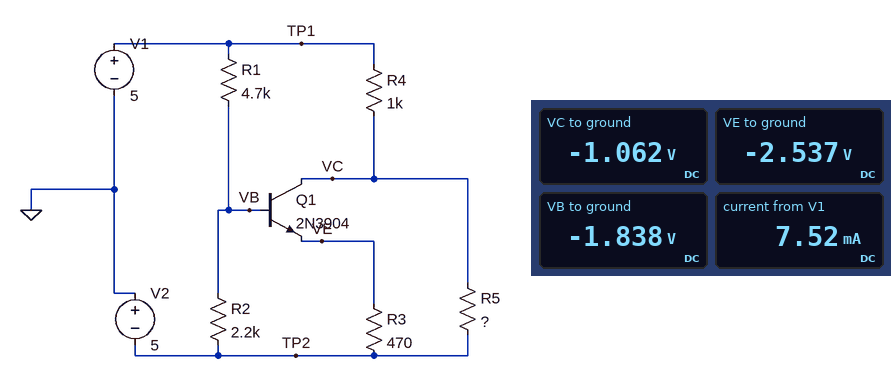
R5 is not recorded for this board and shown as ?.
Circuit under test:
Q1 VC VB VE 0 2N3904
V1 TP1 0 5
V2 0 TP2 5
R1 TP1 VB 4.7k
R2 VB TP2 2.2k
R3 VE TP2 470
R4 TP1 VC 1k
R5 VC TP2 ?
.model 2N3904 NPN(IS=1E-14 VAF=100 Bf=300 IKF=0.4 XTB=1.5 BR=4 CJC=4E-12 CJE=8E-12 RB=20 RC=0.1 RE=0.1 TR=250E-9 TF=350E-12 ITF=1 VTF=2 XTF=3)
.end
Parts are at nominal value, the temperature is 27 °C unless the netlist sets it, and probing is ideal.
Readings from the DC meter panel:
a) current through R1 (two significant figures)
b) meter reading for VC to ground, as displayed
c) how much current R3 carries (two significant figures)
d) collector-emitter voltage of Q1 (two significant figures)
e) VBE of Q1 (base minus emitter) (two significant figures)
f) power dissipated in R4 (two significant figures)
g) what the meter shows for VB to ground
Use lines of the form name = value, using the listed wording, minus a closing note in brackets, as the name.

current through R1 = 1.5 mA
meter reading for VC to ground, as displayed = -1.062 V
how much current R3 carries = 5.2 mA
collector-emitter voltage of Q1 = 1.5 V
VBE of Q1 (base minus emitter) = 700 mV
power dissipated in R4 = 37 mW
what the meter shows for VB to ground = -1.838 V
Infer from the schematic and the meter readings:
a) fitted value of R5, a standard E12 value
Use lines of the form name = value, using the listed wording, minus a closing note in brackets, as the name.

fitted value of R5, a standard E12 value = 4.7 kΩ
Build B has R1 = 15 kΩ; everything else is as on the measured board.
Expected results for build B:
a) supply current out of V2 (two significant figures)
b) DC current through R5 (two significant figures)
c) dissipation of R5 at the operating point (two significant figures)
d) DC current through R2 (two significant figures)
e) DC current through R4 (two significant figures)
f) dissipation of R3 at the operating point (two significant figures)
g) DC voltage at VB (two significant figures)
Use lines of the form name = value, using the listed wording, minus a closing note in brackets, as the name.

supply current out of V2 = 3.4 mA
DC current through R5 = 1.5 mA
dissipation of R5 at the operating point = 11 mW
DC current through R2 = 580 µA
DC current through R4 = 2.8 mA
dissipation of R3 at the operating point = 790 µW
DC voltage at VB = -3.7 V
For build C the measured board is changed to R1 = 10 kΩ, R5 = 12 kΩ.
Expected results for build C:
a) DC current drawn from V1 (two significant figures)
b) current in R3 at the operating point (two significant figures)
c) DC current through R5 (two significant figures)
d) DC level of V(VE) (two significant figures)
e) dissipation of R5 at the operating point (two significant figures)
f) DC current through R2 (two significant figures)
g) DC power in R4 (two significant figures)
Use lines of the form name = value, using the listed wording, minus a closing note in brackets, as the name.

DC current drawn from V1 = 3.8 mA
current in R3 at the operating point = 2.4 mA
DC current through R5 = 590 µA
DC level of V(VE) = -3.9 V
dissipation of R5 at the operating point = 4.1 mW
DC current through R2 = 810 µA
DC power in R4 = 8.7 mW
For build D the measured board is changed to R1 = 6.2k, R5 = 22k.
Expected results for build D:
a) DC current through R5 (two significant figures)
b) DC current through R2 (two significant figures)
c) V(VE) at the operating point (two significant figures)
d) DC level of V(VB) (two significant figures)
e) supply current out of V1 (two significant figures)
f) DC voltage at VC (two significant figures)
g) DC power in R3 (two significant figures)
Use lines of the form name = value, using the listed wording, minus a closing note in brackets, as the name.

DC current through R5 = 260 µA
DC current through R2 = 1.2 mA
V(VE) at the operating point = -3.1 V
DC level of V(VB) = -2.4 V
supply current out of V1 = 5.5 mA
DC voltage at VC = 700 mV
DC power in R3 = 7.7 mW
